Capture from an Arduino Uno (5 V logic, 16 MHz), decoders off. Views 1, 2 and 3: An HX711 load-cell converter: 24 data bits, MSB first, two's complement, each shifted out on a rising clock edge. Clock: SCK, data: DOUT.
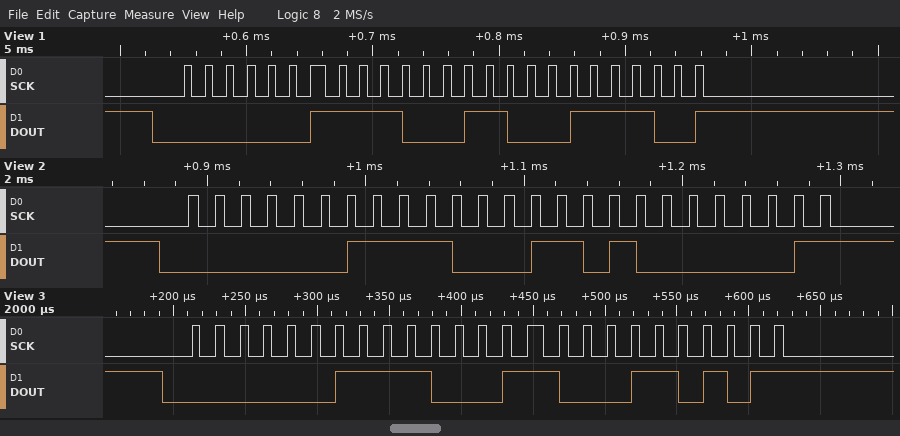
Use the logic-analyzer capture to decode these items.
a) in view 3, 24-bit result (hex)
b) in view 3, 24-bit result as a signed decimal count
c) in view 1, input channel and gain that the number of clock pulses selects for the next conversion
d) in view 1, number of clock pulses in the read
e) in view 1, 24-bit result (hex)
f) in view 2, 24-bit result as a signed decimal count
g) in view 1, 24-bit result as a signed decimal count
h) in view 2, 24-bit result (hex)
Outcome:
0x03C635
247349
channel A, gain 128
25
0x03C63C
247425
247356
0x03C681
